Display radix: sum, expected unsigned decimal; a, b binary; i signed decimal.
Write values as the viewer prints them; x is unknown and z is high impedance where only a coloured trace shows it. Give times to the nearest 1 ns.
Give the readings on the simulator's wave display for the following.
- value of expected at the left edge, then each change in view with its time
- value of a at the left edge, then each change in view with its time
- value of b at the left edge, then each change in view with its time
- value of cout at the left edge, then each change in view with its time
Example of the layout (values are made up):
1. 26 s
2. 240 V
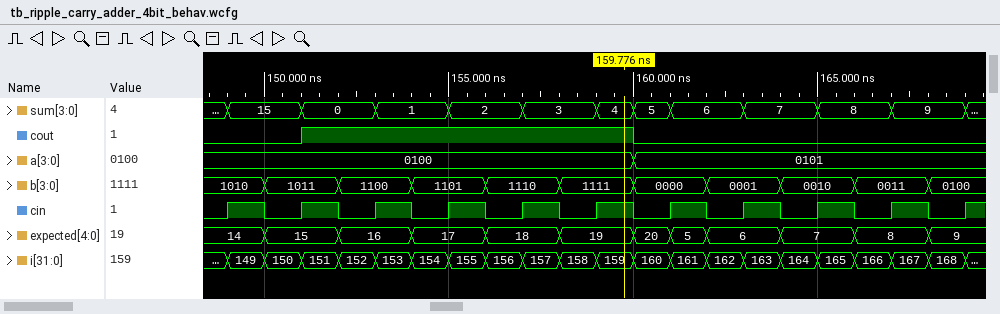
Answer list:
1. 14, 15 at 150 ns, 16 at 152 ns, 17 at 154 ns, 18 at 156 ns, 19 at 158 ns, 20 at 160 ns, 5 at 161 ns, 6 at 162 ns, 7 at 164 ns, 8 at 166 ns, 9 at 168 ns
2. 0100, 0101 at 160 ns
3. 1010, 1011 at 150 ns, 1100 at 152 ns, 1101 at 154 ns, 1110 at 156 ns, 1111 at 158 ns, 0000 at 160 ns, 0001 at 162 ns, 0010 at 164 ns, 0011 at 166 ns, 0100 at 168 ns
4. 0, 1 at 151 ns, 0 at 160 ns
